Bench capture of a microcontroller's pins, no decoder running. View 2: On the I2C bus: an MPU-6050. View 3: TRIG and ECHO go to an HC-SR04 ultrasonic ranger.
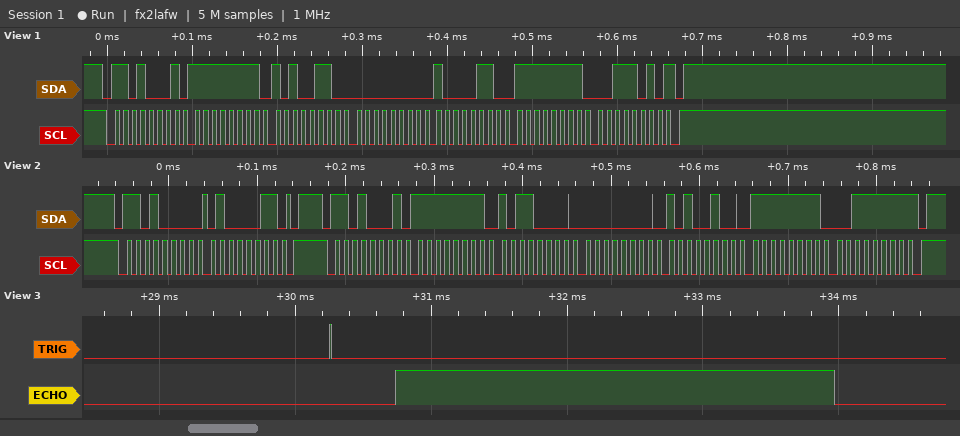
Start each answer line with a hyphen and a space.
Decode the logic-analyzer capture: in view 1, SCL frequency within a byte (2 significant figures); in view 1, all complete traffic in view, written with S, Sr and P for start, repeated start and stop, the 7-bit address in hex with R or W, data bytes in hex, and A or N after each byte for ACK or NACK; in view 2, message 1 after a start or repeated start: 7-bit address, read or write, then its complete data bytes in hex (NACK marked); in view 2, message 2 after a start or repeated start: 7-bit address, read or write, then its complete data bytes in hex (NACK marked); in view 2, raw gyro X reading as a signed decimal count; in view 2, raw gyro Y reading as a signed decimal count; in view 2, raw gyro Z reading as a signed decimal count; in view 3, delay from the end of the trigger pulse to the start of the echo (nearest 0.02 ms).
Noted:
- 100 kHz
- S 68R A FF A A6 A 00 A 86 A FF A 3A N P
- 0x68 write: 43
- 0x68 read: FF B0 00 A4 FF 3F NACK
- -80
- 164
- -193
- 0.46 ms
